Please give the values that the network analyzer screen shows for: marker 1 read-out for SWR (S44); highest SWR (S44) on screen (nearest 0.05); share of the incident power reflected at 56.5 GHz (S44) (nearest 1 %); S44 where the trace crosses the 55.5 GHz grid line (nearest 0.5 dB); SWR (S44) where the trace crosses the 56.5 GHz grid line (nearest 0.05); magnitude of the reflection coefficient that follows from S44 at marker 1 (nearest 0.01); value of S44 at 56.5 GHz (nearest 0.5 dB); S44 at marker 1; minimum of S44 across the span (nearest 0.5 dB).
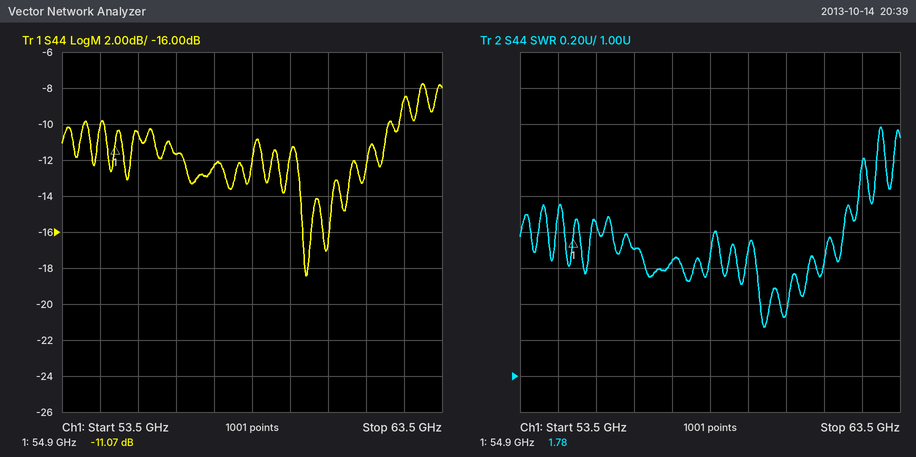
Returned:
1.78
2.40
7 %
-10.5 dB
1.70
0.28
-11.5 dB
-11.07 dB
-18.5 dB
